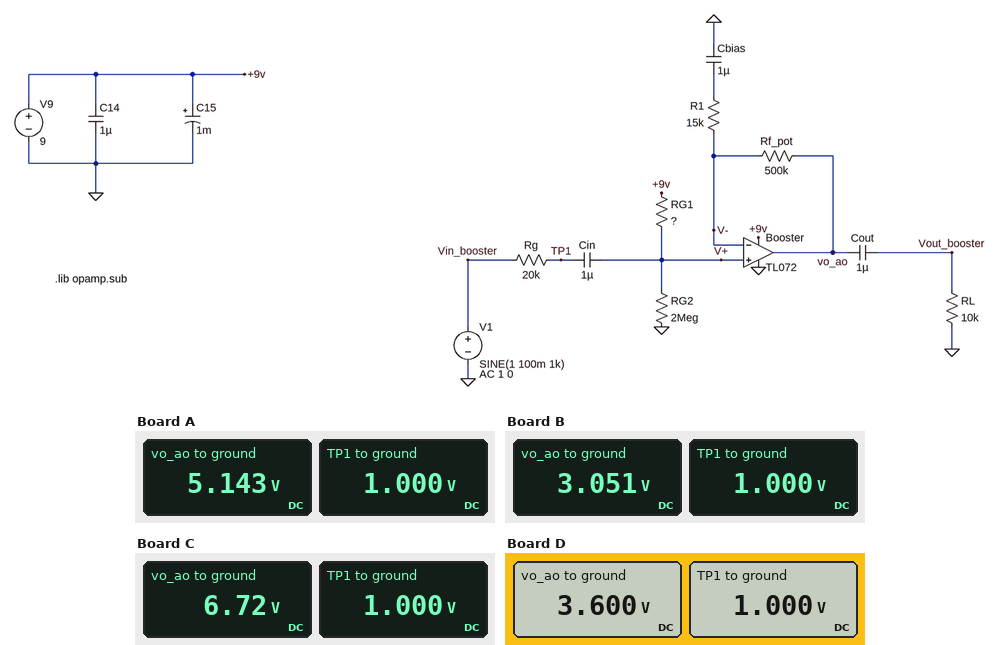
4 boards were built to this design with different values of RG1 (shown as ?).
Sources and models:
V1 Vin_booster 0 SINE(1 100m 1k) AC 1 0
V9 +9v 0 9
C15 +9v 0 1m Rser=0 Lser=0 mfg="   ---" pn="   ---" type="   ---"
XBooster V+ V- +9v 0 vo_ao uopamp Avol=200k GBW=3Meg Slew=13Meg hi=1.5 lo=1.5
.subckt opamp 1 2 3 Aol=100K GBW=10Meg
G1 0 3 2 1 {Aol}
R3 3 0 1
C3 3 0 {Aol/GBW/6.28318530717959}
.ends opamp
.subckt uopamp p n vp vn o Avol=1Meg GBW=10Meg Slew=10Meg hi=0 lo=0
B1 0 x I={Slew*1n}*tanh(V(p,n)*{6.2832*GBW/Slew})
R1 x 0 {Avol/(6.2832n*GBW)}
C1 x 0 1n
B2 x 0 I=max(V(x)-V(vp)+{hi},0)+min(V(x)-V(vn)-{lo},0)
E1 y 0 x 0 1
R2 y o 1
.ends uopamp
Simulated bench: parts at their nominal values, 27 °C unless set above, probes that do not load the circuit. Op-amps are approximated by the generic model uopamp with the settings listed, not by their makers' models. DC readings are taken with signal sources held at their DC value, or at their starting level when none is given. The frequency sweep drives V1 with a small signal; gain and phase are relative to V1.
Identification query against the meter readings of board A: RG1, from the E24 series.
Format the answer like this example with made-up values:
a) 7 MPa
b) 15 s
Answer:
a) 1.5 MΩ
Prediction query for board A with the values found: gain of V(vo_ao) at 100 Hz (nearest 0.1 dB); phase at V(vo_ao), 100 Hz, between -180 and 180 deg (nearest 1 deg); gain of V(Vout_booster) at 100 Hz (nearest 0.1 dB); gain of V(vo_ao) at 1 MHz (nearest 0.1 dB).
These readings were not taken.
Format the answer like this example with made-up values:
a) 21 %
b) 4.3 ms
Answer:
a) 30.5 dB
b) 6 deg
c) 30.4 dB
d) 9.3 dB
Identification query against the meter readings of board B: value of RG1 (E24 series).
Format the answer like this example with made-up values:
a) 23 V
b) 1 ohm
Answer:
a) 3.9 MΩ
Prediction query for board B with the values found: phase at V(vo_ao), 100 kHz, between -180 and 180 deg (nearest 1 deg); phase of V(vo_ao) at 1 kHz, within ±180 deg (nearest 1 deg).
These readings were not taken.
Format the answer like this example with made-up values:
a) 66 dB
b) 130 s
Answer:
a) -49 deg
b) 0 deg
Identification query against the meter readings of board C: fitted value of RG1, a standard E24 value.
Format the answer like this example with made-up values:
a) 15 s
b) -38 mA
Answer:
a) 680 kΩ
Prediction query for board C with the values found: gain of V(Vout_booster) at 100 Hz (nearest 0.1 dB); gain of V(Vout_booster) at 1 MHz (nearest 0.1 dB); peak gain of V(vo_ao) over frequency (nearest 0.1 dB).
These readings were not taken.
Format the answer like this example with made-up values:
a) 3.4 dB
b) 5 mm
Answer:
a) 30.2 dB
b) 9.2 dB
c) 30.4 dB
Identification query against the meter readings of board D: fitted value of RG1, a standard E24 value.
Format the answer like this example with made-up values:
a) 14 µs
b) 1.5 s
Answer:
a) 3 MΩ
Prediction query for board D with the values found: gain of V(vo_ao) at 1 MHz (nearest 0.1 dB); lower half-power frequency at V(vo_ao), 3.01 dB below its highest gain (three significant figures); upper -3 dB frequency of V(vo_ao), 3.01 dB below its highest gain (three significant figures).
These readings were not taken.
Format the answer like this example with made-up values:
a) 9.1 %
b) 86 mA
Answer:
a) 9.4 dB
b) 10.6 Hz
c) 87.4 kHz
